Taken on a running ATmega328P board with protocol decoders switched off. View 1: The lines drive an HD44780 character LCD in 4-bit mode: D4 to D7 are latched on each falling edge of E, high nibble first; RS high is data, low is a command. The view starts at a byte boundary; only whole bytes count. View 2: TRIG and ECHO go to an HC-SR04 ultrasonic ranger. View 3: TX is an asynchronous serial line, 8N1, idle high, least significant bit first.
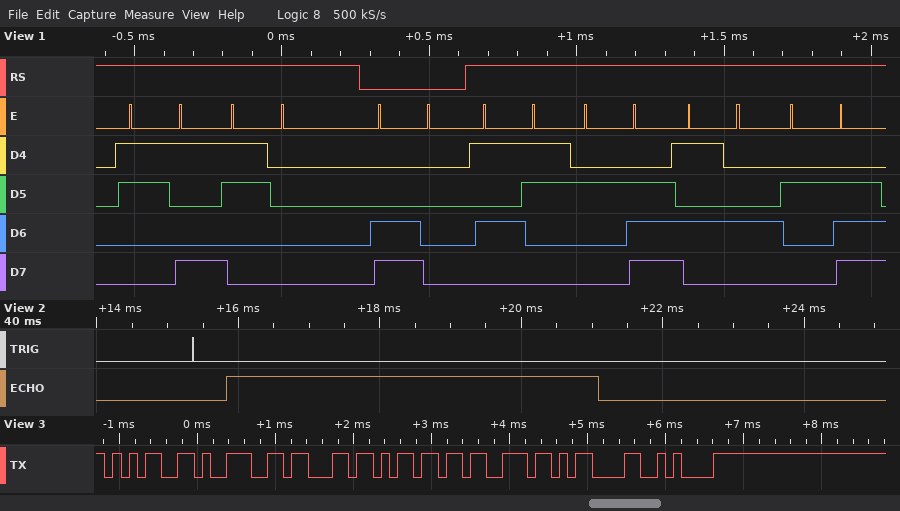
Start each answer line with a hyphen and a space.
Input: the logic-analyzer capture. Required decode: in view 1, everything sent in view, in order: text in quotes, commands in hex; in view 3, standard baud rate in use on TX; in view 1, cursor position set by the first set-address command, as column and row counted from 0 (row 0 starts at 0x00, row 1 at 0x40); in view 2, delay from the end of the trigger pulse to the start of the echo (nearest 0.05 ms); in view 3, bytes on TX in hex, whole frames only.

- "90" 0xC0 "S.T."
- 9600 baud
- column 0, row 1
- 0.45 ms
- 35 39 63 6D 73 0D 0A
